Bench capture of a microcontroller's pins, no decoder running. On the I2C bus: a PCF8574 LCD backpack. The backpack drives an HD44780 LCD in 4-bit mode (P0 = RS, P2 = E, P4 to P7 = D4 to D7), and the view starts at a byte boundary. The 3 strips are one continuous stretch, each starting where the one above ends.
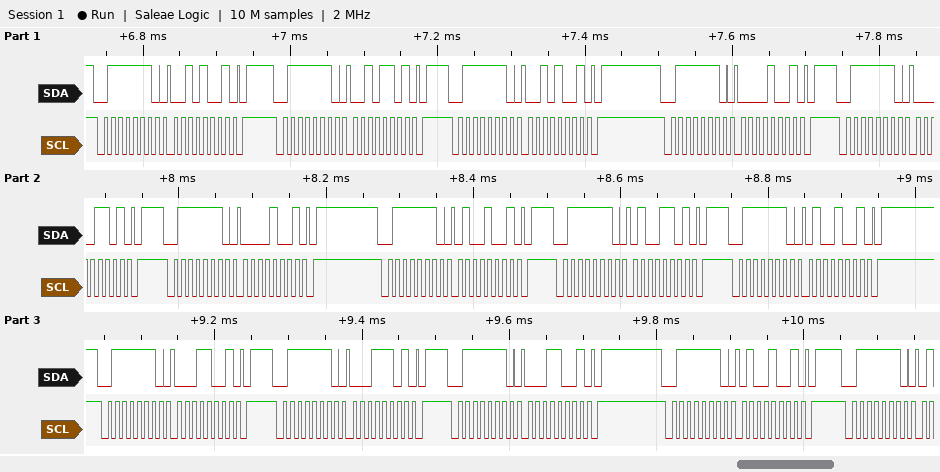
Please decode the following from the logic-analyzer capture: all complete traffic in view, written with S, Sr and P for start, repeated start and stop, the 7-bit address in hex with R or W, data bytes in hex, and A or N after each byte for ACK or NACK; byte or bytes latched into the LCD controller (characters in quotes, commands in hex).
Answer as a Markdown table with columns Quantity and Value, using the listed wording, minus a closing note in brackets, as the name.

| Quantity | Value |
|---|---|
| all complete traffic in view, written with S, Sr and P for start, repeated start and stop, the 7-bit address in hex with R or W, data bytes in hex, and A or N after each byte for ACK or NACK | S 3FW A 29 A P S 3FW A 2D A P S 3FW A 29 A P S 3FW A 09 A P S 3FW A 0D A P S 3FW A 09 A P S 3FW A 49 A P S 3FW A 4D A P S 3FW A 49 A P S 3FW A 19 A P S 3FW A 1D A P S 3FW A 19 A P S 3FW A 49 A P S 3FW A |
| byte or bytes latched into the LCD controller | ' ' 'A' |
